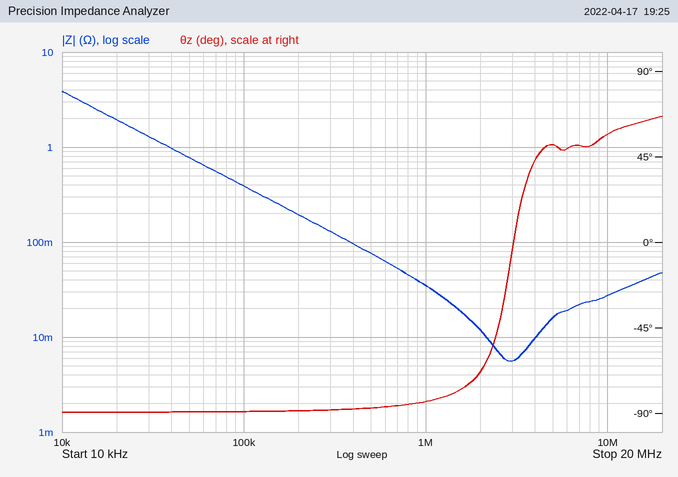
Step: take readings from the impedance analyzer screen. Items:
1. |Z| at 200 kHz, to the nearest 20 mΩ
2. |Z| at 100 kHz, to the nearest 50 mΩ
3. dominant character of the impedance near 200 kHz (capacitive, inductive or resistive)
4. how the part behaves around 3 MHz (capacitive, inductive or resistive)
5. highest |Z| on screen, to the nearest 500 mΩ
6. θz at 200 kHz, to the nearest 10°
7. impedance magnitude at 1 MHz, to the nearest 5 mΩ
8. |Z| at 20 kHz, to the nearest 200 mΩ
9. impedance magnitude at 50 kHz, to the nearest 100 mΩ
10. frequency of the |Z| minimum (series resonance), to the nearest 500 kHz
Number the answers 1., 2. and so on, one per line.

1. 200 mΩ
2. 400 mΩ
3. capacitive
4. resistive
5. 4.0 Ω
6. -90°
7. 35 mΩ
8. 2.0 Ω
9. 800 mΩ
10. 3.0 MHz
